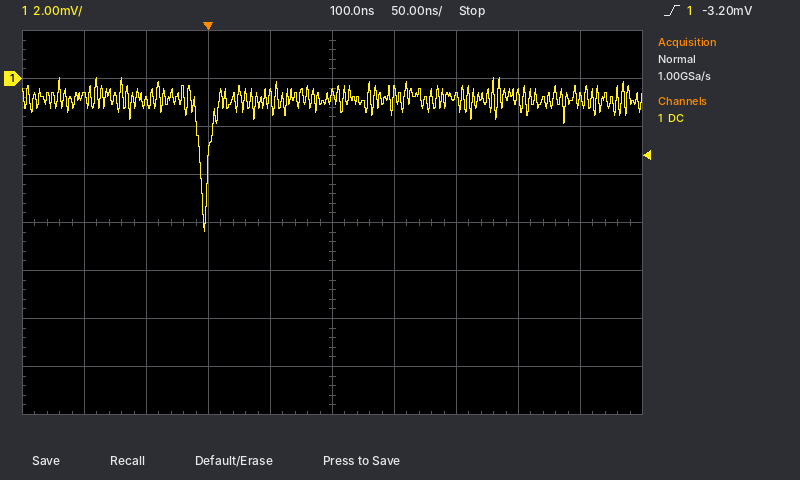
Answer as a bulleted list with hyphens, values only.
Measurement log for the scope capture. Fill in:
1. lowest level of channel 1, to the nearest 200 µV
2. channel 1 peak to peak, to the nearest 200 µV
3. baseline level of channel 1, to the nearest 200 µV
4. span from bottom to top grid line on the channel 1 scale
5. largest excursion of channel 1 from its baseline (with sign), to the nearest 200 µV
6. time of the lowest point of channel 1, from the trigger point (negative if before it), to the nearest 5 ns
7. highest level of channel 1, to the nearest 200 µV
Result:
- -6.4 mV
- 6.4 mV
- -800 µV
- 16 mV
- -5.6 mV
- -5 ns
- 0.0 mV
